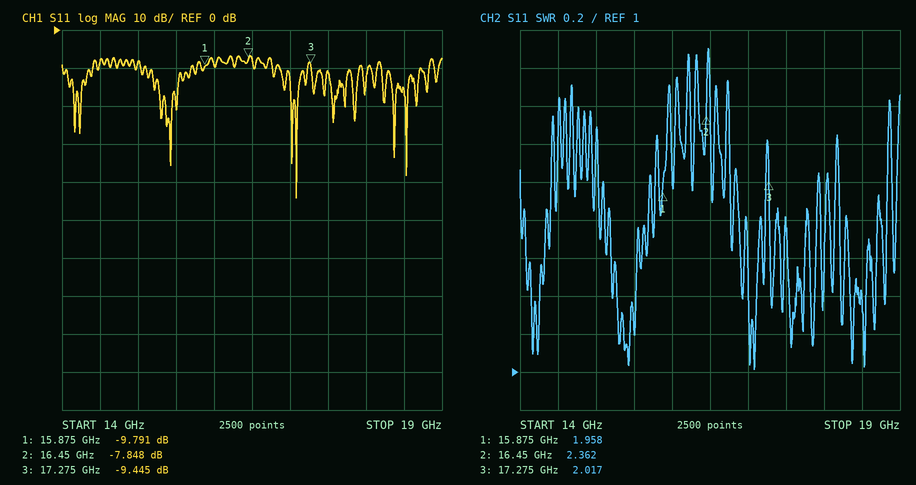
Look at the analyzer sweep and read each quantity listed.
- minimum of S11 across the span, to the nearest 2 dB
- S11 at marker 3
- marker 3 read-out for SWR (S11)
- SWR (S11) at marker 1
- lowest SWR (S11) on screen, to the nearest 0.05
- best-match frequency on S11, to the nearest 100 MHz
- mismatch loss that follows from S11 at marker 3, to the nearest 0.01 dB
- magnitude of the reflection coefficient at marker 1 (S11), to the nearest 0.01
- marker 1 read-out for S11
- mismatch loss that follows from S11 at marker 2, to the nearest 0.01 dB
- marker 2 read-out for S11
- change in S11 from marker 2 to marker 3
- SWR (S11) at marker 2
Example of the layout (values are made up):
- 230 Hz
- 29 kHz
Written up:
- -44 dB
- -9.445 dB
- 2.017
- 1.958
- 1.00
- 17.1 GHz
- 0.52 dB
- 0.32
- -9.791 dB
- 0.78 dB
- -7.848 dB
- -1.597 dB
- 2.362
